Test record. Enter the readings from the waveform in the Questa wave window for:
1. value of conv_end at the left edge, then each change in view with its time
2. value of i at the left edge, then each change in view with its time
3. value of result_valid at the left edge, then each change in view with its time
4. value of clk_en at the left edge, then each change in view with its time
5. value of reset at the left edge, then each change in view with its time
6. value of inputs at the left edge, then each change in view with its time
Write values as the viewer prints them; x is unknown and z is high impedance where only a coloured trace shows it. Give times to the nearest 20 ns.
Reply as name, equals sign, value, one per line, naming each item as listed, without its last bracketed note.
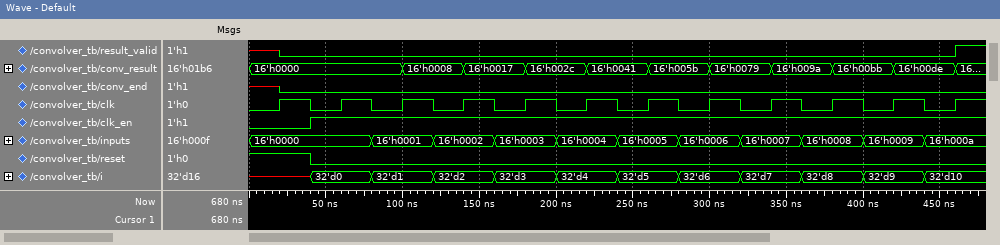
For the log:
value of conv_end at the left edge, then each change in view with its time = x, 0 at 20 ns
value of i at the left edge, then each change in view with its time = x, 32'd0 at 40 ns, 32'd1 at 80 ns, 32'd2 at 120 ns, 32'd3 at 160 ns, 32'd4 at 200 ns, 32'd5 at 240 ns, 32'd6 at 280 ns, 32'd7 at 320 ns, 32'd8 at 360 ns, 32'd9 at 400 ns, 32'd10 at 440 ns
value of result_valid at the left edge, then each change in view with its time = x, 0 at 20 ns, 1 at 460 ns
value of clk_en at the left edge, then each change in view with its time = 0, 1 at 40 ns
value of reset at the left edge, then each change in view with its time = 1, 0 at 40 ns
value of inputs at the left edge, then each change in view with its time = 16'h0000, 16'h0001 at 80 ns, 16'h0002 at 120 ns, 16'h0003 at 160 ns, 16'h0004 at 200 ns, 16'h0005 at 240 ns, 16'h0006 at 280 ns, 16'h0007 at 320 ns, 16'h0008 at 360 ns, 16'h0009 at 400 ns, 16'h000a at 440 ns
